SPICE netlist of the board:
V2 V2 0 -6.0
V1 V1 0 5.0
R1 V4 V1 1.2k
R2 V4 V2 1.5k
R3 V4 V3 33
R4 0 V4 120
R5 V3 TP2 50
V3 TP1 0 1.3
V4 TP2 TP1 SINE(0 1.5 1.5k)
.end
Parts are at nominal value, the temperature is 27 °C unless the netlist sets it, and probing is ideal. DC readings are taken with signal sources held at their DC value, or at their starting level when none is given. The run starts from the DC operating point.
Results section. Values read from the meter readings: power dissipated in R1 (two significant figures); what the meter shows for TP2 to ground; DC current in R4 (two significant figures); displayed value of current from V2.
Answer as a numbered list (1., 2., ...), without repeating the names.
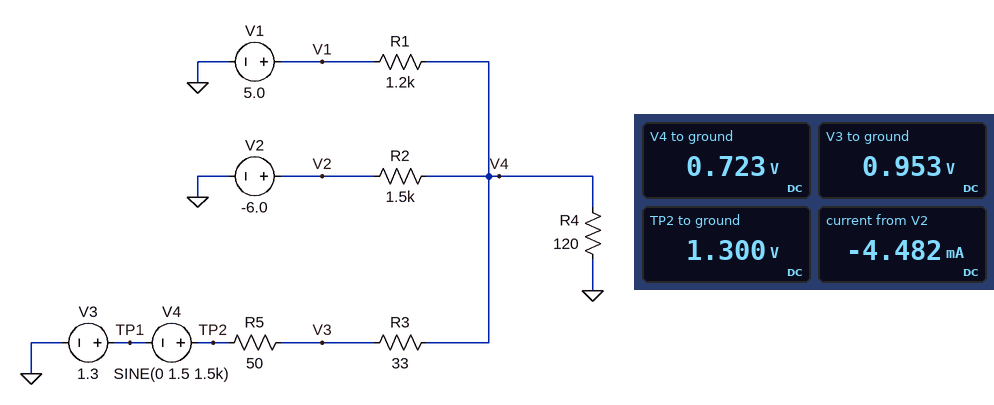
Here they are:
1. 15 mW
2. 1.300 V
3. 6.0 mA
4. -4.482 mA
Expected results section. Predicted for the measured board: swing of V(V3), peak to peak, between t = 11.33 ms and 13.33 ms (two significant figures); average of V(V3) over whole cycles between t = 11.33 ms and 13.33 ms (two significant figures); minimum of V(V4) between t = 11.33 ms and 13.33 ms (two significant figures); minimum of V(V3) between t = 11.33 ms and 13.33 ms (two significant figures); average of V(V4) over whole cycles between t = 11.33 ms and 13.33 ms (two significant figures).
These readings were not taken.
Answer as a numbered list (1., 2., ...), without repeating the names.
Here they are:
1. 2.2 V
2. 950 mV
3. -100 mV
4. -140 mV
5. 720 mV
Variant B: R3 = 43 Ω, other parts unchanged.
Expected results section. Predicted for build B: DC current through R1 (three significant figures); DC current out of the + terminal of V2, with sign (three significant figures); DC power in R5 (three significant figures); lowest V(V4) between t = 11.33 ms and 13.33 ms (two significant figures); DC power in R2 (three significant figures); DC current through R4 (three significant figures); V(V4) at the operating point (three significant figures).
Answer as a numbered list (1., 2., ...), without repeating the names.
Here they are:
1. 3.59 mA
2. -4.46 mA
3. 2.17 mW
4. -96 mV
5. 29.8 mW
6. 5.73 mA
7. 687 mV
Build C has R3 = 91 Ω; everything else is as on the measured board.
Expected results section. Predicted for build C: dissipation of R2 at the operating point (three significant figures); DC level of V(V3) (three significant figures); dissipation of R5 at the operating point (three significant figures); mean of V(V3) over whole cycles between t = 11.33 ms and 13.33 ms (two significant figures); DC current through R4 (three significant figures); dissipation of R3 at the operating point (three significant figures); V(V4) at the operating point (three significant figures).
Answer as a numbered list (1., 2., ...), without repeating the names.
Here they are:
1. 28.6 mW
2. 1.04 V
3. 1.40 mW
4. 1.0 V
5. 4.62 mA
6. 2.54 mW
7. 555 mV
